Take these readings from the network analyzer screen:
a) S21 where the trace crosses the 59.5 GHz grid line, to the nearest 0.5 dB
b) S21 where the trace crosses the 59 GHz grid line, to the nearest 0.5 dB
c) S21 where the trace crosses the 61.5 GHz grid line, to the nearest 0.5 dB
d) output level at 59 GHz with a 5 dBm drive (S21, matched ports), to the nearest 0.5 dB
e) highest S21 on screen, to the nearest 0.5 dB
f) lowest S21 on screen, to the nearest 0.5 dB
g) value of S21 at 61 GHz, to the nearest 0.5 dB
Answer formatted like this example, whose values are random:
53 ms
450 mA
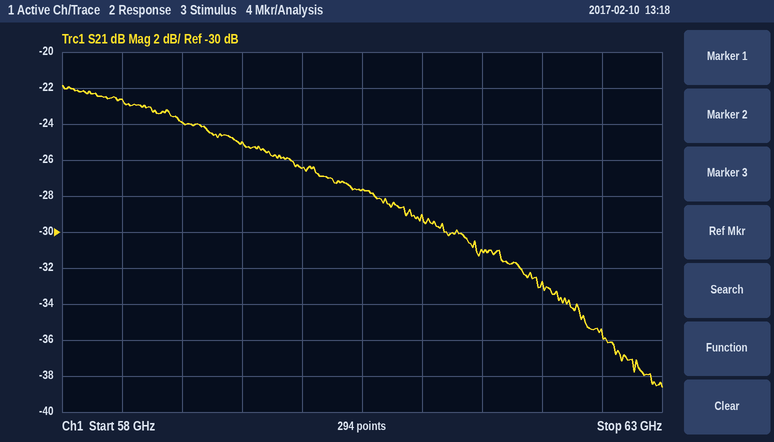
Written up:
-25.0 dB
-24.0 dB
-31.0 dB
-19.0 dBm
-22.0 dB
-38.5 dB
-29.0 dB
